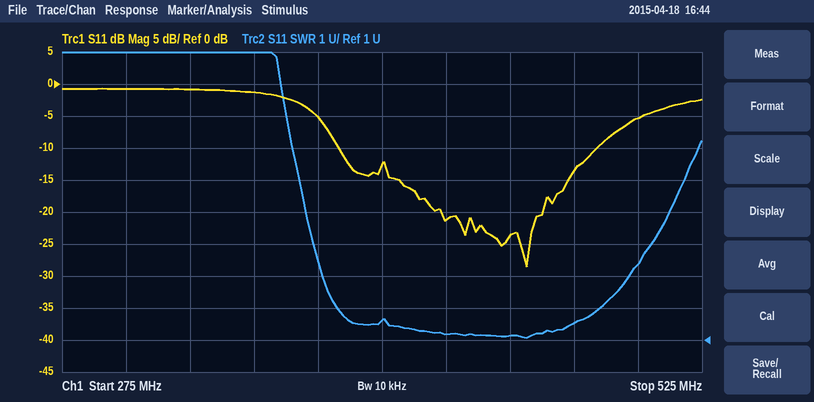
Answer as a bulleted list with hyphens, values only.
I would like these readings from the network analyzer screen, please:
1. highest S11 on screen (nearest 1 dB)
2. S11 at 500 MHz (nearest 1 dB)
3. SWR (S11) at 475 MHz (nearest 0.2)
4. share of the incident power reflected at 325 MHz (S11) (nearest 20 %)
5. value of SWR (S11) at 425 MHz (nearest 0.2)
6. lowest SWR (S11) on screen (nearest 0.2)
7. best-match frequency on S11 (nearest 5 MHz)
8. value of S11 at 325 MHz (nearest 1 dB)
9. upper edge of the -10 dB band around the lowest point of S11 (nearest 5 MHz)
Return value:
- -1 dB
- -5 dB
- 1.6
- 80 %
- 1.2
- 1.0
- 455 MHz
- -1 dB
- 485 MHz
